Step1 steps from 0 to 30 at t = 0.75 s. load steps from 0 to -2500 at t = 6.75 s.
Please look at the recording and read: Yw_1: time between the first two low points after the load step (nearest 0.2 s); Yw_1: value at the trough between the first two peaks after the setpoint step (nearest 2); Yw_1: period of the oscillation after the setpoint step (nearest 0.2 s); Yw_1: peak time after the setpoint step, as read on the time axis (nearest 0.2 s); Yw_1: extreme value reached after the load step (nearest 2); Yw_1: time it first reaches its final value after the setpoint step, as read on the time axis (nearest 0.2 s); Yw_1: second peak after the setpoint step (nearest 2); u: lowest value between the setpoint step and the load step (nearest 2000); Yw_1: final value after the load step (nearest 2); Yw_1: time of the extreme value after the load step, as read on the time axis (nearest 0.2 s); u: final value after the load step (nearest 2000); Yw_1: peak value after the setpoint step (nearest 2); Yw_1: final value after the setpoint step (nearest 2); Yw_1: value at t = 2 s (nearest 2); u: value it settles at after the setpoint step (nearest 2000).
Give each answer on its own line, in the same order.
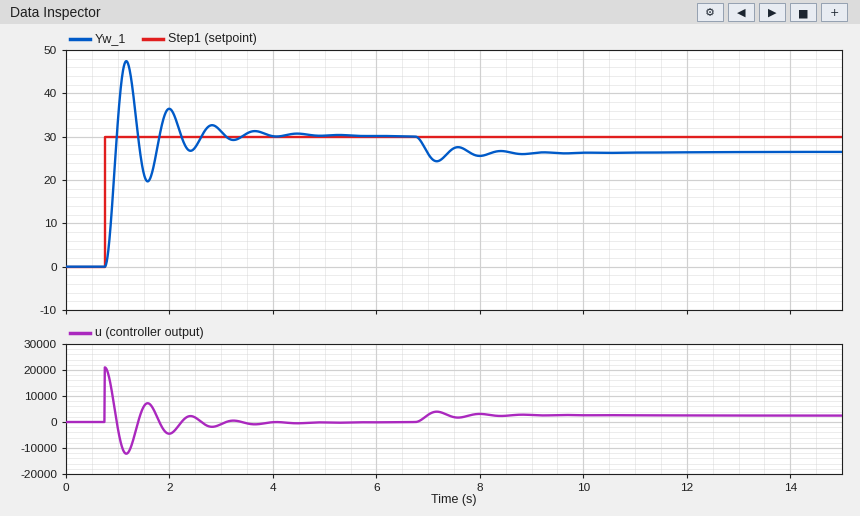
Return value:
0.8 s
20
0.8 s
1.2 s
24
1.0 s
36
-12000
26
7.2 s
2000
48
30
36
0
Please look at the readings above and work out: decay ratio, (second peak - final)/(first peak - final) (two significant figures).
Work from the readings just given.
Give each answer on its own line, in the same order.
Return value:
0.33
